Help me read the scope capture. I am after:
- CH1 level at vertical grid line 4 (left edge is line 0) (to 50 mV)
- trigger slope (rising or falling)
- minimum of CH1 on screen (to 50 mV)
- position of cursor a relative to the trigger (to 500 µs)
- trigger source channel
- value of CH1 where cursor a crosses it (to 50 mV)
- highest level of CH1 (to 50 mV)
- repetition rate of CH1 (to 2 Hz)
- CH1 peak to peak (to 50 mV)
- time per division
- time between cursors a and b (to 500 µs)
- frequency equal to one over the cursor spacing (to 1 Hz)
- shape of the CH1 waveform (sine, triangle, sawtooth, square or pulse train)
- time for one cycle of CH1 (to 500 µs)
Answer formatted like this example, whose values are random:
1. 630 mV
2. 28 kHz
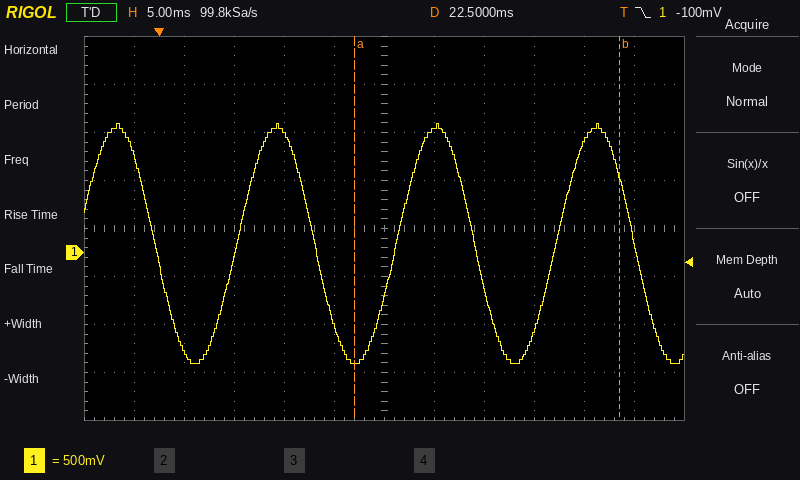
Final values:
1. 1.25 V
2. falling
3. -1.15 V
4. +19.5 ms
5. CH1
6. -1.15 V
7. 1.35 V
8. 62 Hz
9. 2.50 V
10. 5 ms
11. 26.5 ms
12. 38 Hz
13. sine
14. 16.0 ms
